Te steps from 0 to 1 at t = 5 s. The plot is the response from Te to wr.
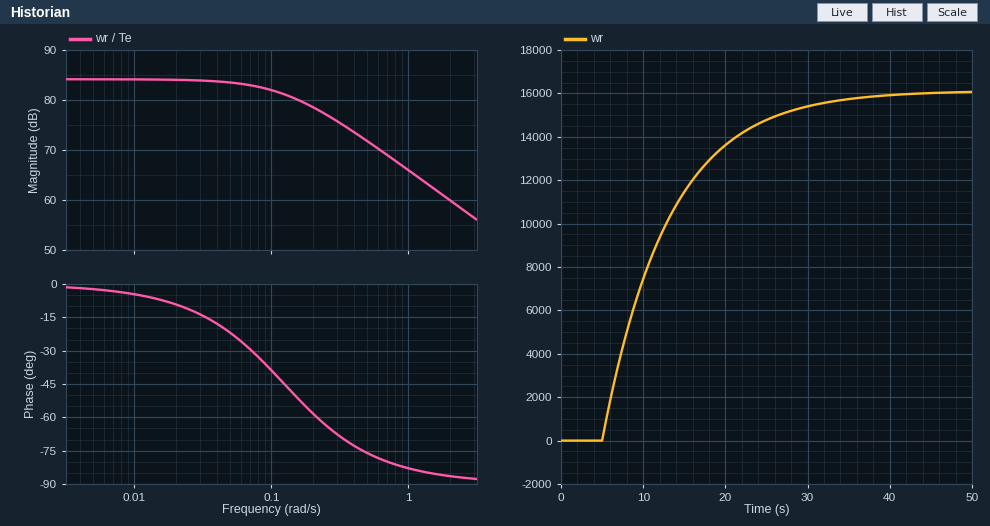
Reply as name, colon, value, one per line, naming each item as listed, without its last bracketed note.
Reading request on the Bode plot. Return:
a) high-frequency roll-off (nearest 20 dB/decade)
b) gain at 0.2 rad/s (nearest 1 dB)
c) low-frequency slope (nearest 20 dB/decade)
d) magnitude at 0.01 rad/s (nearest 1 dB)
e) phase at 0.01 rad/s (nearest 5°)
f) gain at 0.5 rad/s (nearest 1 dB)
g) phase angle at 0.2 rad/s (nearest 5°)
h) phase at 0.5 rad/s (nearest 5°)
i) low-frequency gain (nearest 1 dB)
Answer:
high-frequency roll-off: -20 dB/decade
gain at 0.2 rad/s: 79 dB
low-frequency slope: 0 dB/decade
magnitude at 0.01 rad/s: 84 dB
phase at 0.01 rad/s: -5°
gain at 0.5 rad/s: 72 dB
phase angle at 0.2 rad/s: -60°
phase at 0.5 rad/s: -75°
low-frequency gain: 84 dB
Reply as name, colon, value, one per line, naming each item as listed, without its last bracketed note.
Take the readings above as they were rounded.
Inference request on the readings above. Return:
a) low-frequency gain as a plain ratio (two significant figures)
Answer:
low-frequency gain as a plain ratio: 16000
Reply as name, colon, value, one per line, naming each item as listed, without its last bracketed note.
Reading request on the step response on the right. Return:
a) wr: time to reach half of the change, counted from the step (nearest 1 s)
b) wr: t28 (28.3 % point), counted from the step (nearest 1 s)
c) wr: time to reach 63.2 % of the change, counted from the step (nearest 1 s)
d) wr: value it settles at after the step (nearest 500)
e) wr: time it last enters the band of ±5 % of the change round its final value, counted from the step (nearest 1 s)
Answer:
wr: time to reach half of the change, counted from the step: 6 s
wr: t28 (28.3 % point), counted from the step: 3 s
wr: time to reach 63.2 % of the change, counted from the step: 8 s
wr: value it settles at after the step: 16000
wr: time it last enters the band of ±5 % of the change round its final value, counted from the step: 24 s
